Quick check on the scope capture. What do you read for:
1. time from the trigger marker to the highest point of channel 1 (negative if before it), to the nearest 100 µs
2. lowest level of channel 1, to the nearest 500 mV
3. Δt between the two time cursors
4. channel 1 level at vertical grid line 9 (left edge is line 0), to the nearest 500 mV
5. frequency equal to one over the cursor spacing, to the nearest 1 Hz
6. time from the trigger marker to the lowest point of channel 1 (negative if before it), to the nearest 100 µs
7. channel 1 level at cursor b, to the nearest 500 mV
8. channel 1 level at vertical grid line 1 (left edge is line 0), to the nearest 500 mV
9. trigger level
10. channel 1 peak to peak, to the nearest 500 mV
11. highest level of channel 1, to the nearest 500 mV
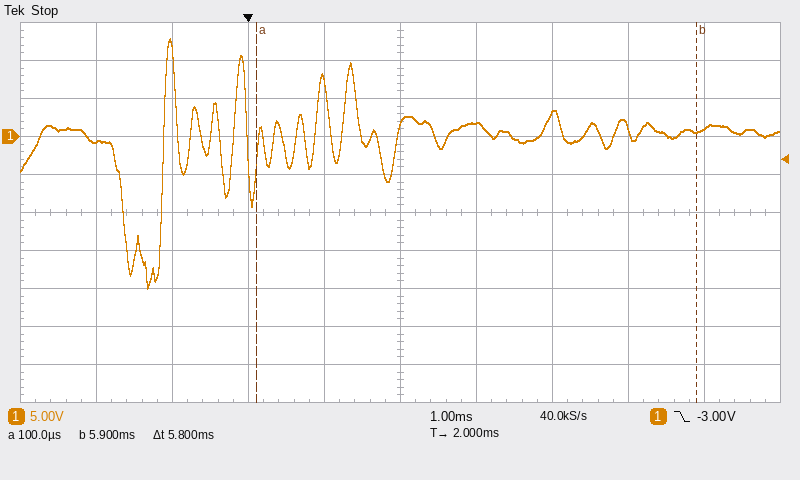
-1.0 ms
-20.0 V
5.8 ms
1.0 V
172 Hz
-1.3 ms
500 mV
-500 mV
-3.00 V
33.0 V
13.0 V
